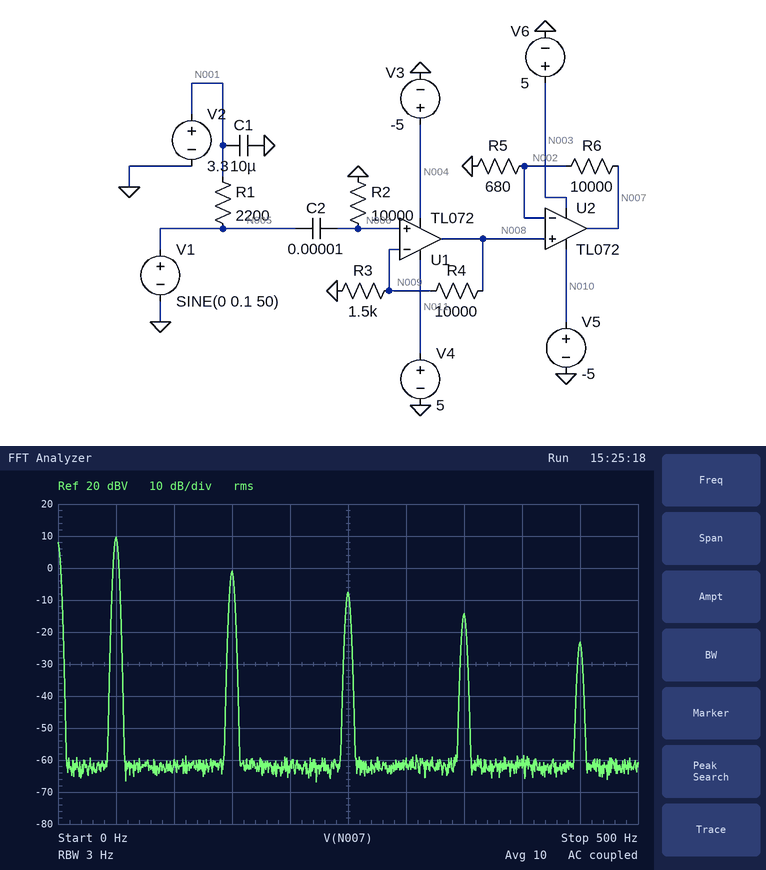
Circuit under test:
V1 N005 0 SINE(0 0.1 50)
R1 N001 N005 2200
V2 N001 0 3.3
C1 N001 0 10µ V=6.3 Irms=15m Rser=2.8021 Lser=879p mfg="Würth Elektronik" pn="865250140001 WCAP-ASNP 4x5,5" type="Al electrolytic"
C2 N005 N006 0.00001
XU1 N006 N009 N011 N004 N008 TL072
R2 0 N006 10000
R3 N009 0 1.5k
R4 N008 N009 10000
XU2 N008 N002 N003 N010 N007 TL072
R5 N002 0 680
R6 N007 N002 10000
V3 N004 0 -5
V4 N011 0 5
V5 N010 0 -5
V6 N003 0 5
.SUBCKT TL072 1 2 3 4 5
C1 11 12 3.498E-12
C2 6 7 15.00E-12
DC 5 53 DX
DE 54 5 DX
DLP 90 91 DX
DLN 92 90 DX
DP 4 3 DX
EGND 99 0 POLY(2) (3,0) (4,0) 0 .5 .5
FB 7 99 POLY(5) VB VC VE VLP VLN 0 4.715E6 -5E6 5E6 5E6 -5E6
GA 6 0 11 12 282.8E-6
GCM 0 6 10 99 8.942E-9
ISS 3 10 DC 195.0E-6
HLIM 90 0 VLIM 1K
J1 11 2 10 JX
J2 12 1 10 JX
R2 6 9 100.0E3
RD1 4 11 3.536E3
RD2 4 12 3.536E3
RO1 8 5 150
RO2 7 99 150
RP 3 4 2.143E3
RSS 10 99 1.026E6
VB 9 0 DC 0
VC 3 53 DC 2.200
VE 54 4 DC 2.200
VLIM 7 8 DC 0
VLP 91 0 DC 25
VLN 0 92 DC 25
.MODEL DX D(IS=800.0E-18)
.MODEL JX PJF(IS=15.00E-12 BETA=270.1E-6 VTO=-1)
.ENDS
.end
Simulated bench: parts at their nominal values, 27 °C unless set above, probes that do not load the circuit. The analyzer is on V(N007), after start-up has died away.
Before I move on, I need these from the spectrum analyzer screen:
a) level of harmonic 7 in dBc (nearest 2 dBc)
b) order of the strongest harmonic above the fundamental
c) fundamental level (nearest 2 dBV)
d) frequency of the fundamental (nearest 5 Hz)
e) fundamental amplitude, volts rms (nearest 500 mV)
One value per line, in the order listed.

-24 dBc
3
10 dBV
50 Hz
3.0 V
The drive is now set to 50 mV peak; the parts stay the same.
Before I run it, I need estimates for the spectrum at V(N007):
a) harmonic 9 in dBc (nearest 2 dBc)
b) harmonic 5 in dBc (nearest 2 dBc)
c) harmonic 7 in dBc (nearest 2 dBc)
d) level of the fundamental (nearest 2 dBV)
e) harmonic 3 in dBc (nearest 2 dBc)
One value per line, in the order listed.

-36 dBc
-36 dBc
-32 dBc
10 dBV
-14 dBc
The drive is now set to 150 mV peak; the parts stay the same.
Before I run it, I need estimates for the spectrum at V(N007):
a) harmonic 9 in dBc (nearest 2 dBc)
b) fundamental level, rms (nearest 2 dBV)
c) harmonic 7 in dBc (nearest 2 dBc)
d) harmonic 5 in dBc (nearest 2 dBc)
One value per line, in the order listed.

-24 dBc
10 dBV
-20 dBc
-16 dBc
